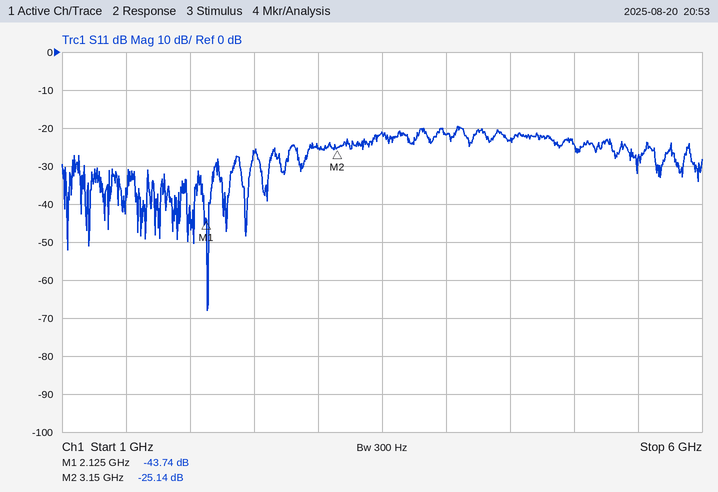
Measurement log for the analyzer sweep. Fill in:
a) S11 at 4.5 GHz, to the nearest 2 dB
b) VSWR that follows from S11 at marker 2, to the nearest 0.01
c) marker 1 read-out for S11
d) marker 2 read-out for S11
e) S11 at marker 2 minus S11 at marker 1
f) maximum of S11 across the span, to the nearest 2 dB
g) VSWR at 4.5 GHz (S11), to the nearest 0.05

-24 dB
1.12
-43.74 dB
-25.14 dB
18.60 dB
-20 dB
1.15
